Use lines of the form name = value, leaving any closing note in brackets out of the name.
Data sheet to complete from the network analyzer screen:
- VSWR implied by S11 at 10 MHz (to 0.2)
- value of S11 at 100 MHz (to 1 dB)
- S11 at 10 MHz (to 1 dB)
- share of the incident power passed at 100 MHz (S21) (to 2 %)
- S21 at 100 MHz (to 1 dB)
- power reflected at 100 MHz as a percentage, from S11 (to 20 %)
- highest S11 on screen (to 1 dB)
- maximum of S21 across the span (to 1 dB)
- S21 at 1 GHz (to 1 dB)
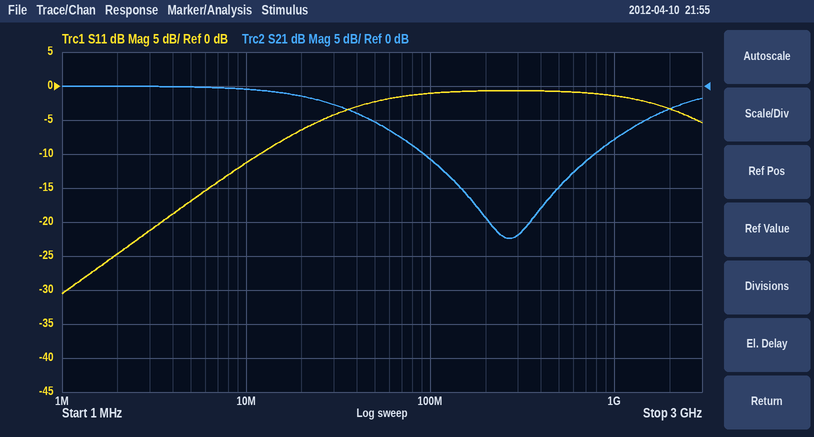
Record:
VSWR implied by S11 at 10 MHz = 1.8
value of S11 at 100 MHz = -1 dB
S11 at 10 MHz = -11 dB
share of the incident power passed at 100 MHz (S21) = 8 %
S21 at 100 MHz = -11 dB
power reflected at 100 MHz as a percentage, from S11 = 80 %
highest S11 on screen = -1 dB
maximum of S21 across the span = 0 dB
S21 at 1 GHz = -8 dB
